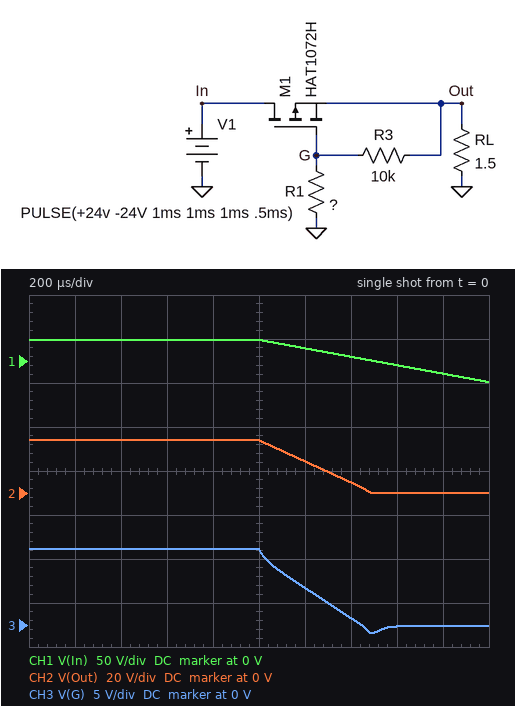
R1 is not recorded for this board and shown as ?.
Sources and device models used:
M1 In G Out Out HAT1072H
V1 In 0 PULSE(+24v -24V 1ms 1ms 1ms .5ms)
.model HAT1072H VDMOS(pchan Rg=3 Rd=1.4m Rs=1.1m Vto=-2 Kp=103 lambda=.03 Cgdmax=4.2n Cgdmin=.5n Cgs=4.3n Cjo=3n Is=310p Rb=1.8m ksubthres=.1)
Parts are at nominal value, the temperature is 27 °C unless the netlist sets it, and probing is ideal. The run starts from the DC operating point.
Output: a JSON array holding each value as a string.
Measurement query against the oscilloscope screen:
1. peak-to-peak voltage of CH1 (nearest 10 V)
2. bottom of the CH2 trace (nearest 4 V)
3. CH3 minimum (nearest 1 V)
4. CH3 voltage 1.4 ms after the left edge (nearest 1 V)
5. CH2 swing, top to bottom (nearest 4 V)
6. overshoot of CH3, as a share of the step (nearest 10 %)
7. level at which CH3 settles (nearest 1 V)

["50 V", "0 V", "-1 V", "1 V", "24 V", "10 %", "0 V"]
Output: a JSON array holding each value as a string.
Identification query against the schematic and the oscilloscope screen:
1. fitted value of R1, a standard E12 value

["5.6 kΩ"]
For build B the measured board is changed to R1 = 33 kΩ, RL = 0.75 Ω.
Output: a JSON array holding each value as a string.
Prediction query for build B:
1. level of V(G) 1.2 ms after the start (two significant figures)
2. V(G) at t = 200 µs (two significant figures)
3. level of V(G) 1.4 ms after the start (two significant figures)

["10 V", "18 V", "2.6 V"]
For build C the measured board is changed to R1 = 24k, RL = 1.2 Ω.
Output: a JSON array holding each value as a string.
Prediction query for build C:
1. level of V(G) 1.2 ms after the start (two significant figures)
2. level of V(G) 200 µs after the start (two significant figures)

["9.3 V", "17 V"]
